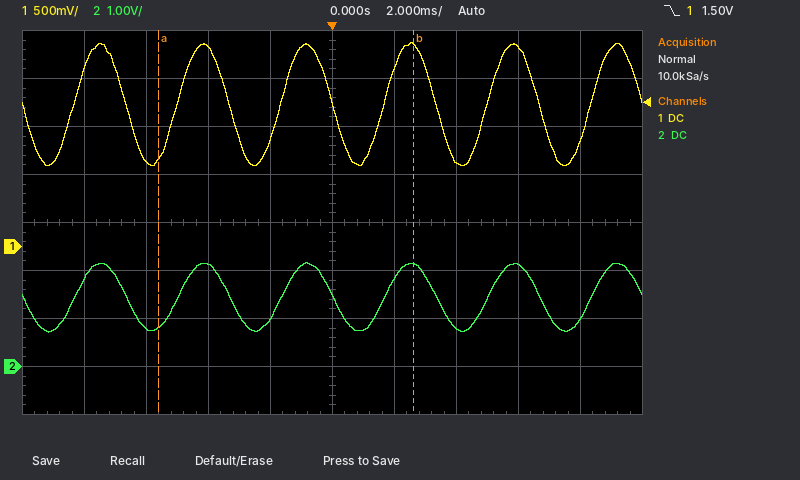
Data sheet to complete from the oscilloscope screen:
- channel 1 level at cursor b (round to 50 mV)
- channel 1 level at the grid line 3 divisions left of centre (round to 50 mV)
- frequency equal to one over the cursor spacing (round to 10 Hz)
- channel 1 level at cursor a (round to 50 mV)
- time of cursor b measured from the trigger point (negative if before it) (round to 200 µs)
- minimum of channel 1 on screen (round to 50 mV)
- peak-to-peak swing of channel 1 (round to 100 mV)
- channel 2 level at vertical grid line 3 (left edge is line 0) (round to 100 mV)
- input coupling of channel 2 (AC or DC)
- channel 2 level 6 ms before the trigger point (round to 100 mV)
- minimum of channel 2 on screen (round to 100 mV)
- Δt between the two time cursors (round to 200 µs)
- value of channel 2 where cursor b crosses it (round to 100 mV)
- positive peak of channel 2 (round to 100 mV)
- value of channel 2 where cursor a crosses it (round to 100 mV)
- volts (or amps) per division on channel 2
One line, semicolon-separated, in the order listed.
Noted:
2.10 V; 900 mV; 120 Hz; 900 mV; +2.6 ms; 850 mV; 1.30 V; 2.1 V; DC; 800 mV; 700 mV; 8.2 ms; 2.1 V; 2.2 V; 800 mV; 1 V
